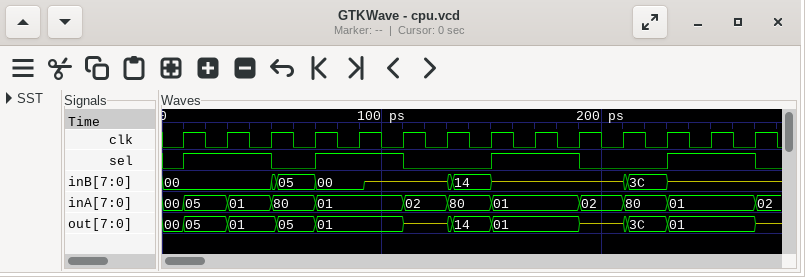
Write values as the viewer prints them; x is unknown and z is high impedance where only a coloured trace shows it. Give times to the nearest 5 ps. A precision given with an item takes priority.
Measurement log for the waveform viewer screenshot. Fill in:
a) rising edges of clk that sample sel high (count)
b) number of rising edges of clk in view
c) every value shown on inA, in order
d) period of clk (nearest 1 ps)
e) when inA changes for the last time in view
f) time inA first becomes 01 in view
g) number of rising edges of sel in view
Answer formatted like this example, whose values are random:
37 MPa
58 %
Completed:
8
14
00, 05, 01, 80, 01, 02, 80, 01, 02, 80, 01, 02
20 ps
270 ps
30 ps
4
